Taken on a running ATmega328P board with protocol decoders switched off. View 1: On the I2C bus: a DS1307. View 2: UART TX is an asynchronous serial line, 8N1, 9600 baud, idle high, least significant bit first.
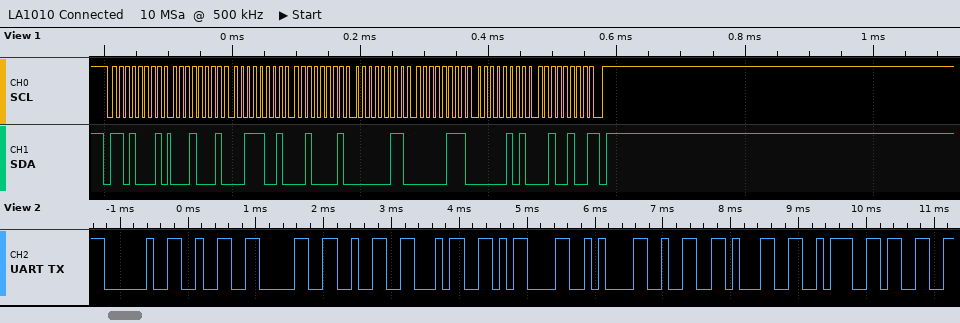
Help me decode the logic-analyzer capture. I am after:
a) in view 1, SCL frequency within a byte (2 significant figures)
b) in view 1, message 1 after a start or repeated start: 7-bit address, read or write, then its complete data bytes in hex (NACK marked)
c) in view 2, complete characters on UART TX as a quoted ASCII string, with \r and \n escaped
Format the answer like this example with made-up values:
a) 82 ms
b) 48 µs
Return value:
a) 100 kHz
b) 0x68 read: 11 39 21 03 07 05 24 NACK
c) " 2024\r\n21:3"
